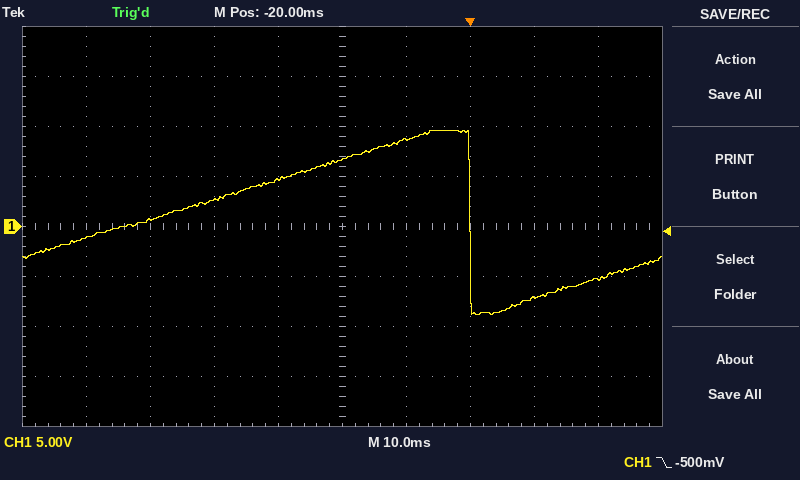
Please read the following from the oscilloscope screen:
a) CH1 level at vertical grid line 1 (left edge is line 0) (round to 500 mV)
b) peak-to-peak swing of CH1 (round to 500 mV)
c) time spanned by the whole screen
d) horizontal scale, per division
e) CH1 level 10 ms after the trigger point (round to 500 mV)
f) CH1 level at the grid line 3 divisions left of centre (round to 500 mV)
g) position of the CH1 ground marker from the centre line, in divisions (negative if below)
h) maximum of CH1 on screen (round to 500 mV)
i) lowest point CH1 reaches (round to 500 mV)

-1.0 V
18.5 V
100 ms
10 ms
-7.0 V
500 mV
0.0 div
9.5 V
-9.0 V
